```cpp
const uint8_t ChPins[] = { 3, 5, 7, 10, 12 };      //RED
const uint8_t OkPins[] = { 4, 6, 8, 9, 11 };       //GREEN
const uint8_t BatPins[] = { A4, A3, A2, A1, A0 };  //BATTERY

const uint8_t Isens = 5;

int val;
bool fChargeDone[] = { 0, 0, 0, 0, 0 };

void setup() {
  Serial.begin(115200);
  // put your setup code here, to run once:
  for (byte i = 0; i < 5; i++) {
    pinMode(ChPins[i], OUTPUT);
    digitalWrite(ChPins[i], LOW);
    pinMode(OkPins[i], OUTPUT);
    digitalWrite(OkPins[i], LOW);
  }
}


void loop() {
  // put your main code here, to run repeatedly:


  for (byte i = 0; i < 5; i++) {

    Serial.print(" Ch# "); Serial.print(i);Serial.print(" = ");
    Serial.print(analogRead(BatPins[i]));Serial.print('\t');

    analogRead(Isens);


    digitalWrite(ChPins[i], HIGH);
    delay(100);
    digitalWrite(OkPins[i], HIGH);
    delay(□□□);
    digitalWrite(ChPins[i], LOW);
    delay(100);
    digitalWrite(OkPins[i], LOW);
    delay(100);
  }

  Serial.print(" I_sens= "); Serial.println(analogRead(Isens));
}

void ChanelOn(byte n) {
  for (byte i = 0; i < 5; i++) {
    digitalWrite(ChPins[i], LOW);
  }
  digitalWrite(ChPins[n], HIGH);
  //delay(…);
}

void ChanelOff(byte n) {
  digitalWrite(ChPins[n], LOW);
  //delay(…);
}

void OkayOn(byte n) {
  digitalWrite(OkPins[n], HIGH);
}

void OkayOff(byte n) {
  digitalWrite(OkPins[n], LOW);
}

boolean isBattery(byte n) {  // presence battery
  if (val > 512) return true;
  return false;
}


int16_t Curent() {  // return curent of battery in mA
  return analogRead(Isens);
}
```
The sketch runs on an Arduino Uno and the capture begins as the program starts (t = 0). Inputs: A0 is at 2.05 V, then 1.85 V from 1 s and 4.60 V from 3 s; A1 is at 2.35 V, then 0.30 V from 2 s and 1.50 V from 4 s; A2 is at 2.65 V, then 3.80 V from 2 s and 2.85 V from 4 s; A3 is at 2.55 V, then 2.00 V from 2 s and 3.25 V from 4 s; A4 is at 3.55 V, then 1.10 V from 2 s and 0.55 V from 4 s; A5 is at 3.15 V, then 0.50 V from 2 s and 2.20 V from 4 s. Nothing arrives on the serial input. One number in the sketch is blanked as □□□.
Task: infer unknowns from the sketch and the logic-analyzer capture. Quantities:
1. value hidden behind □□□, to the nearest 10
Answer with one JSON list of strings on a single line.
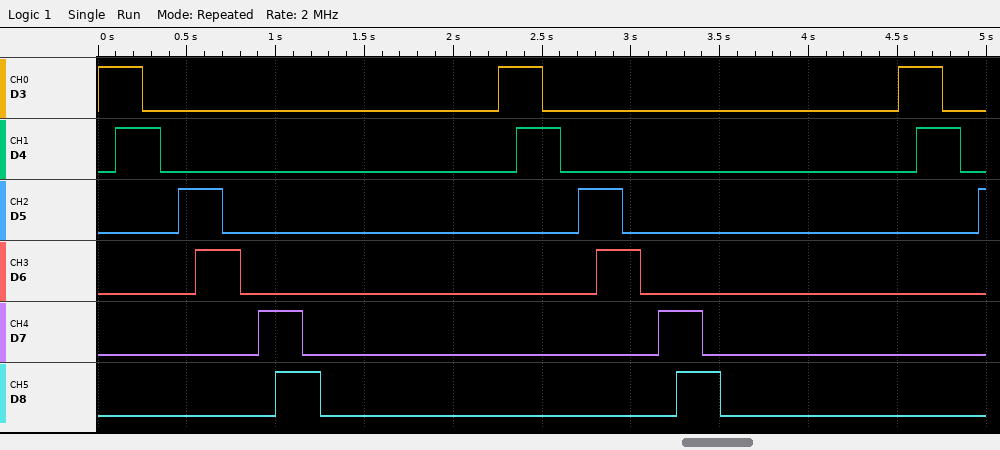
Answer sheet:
["150"]
